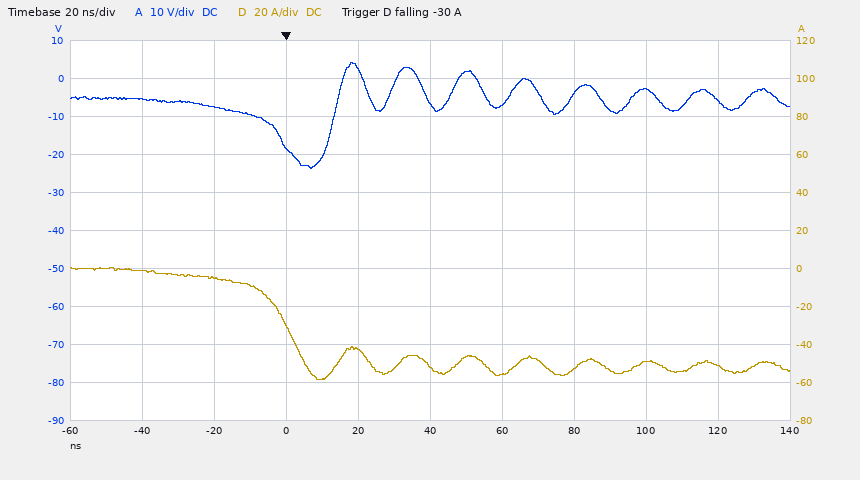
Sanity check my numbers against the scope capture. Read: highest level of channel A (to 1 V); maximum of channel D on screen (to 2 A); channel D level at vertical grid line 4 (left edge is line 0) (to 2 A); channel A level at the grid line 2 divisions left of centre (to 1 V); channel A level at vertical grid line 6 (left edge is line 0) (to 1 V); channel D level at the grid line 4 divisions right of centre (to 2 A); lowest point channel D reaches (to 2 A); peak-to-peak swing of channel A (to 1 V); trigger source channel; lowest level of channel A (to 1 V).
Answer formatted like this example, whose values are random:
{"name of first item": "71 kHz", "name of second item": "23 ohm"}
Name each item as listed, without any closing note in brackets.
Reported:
{"highest level of channel A": "4 V", "maximum of channel D on screen": "0 A", "channel D level at vertical grid line 4 (left edge is line 0)": "-42 A", "channel A level at the grid line 2 divisions left of centre": "-18 V", "channel A level at vertical grid line 6 (left edge is line 0)": "-7 V", "channel D level at the grid line 4 divisions right of centre": "-52 A", "lowest point channel D reaches": "-58 A", "peak-to-peak swing of channel A": "28 V", "trigger source channel": "channel D", "lowest level of channel A": "-24 V"}
